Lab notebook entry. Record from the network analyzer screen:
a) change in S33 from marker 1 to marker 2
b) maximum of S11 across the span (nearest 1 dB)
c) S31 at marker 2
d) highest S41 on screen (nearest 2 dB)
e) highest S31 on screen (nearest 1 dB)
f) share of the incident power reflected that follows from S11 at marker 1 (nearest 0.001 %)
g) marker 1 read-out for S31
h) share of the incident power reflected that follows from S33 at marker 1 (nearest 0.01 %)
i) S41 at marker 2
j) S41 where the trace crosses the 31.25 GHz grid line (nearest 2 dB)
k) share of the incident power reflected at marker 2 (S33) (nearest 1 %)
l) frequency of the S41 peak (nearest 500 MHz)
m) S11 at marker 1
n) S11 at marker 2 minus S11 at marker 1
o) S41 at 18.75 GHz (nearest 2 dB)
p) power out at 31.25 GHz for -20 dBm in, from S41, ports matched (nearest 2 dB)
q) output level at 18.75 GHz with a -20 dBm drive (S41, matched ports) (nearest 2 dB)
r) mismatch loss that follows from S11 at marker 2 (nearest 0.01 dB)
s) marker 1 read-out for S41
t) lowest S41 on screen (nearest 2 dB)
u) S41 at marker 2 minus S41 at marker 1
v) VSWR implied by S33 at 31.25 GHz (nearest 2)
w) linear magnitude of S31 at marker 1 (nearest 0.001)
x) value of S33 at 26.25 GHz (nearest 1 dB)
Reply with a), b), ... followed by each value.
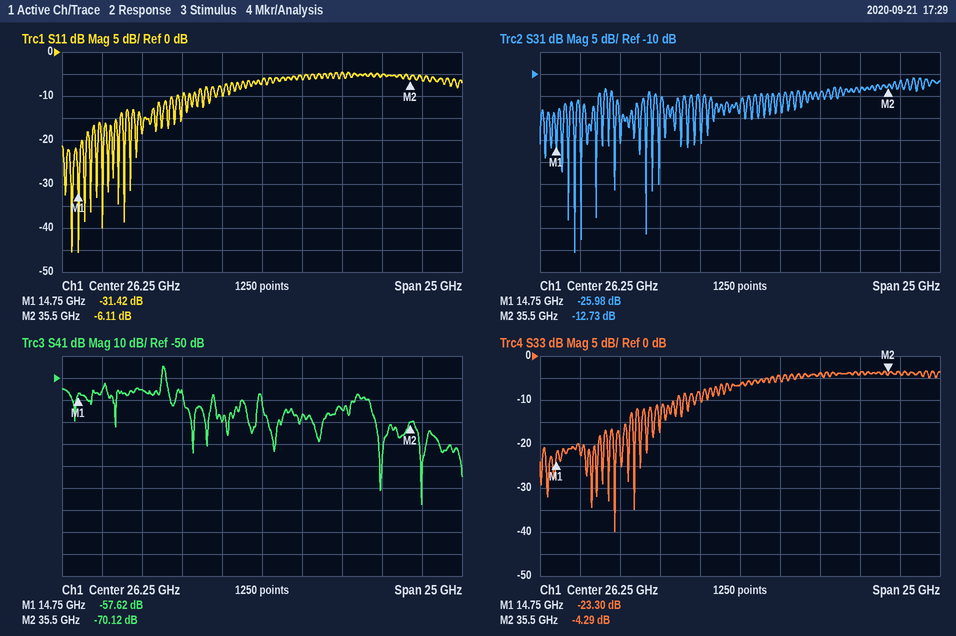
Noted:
a) 19.01 dB
b) -5 dB
c) -12.73 dB
d) -44 dB
e) -11 dB
f) 0.072 %
g) -25.98 dB
h) 0.47 %
i) -70.12 dB
j) -64 dB
k) 37 %
l) 20.0 GHz
m) -31.42 dB
n) 25.31 dB
o) -56 dB
p) -84 dBm
q) -76 dBm
r) 1.22 dB
s) -57.62 dB
t) -108 dB
u) -12.50 dB
v) 4
w) 0.050
x) -7 dB
